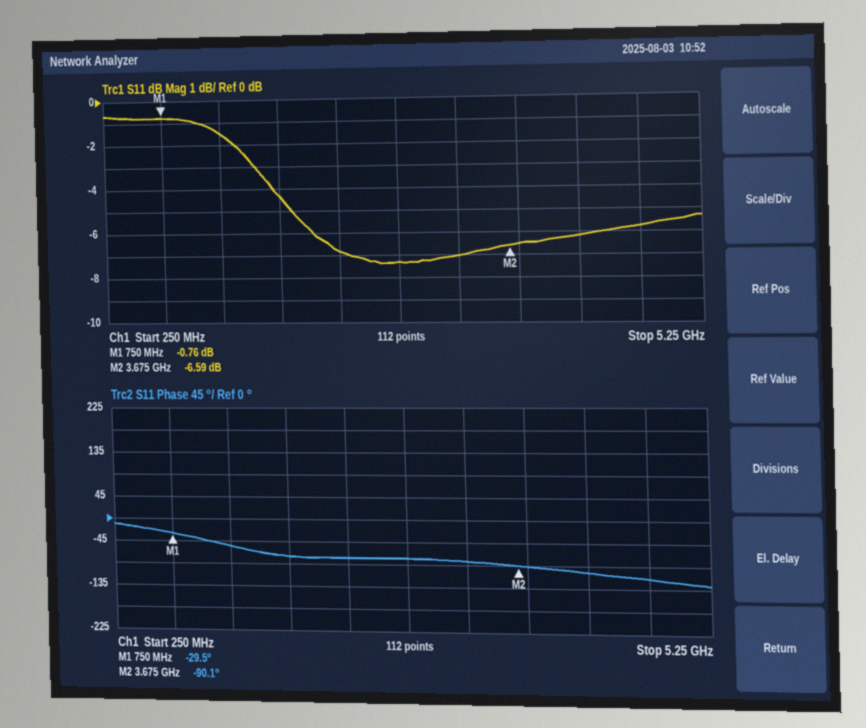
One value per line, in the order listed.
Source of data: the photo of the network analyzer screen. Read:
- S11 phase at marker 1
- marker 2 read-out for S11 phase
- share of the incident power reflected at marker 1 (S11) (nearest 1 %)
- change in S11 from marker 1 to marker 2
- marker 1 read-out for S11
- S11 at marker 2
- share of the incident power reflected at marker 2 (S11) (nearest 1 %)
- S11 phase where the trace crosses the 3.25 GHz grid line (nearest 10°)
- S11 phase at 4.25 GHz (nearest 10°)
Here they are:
-29.5°
-90.1°
84 %
-5.83 dB
-0.76 dB
-6.59 dB
22 %
-80°
-100°
